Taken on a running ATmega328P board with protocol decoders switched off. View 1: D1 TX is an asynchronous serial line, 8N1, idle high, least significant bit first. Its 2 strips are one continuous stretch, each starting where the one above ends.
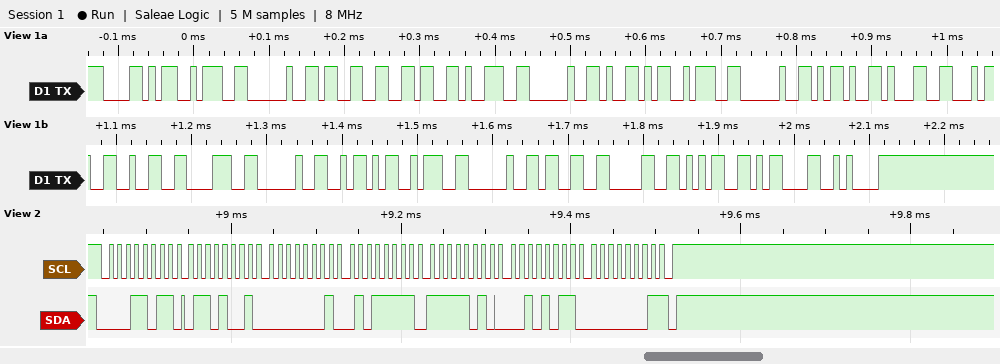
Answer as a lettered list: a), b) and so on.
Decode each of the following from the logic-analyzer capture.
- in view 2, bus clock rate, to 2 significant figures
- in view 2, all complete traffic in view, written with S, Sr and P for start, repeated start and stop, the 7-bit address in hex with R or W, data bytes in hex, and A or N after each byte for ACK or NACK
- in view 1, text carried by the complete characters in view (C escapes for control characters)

a) 100 kHz
b) S 0DR A 69 A 01 A 5F A FA A 2B A 01 N P
c) "X: 369 Y: -1428 Z: 305\r\n"
